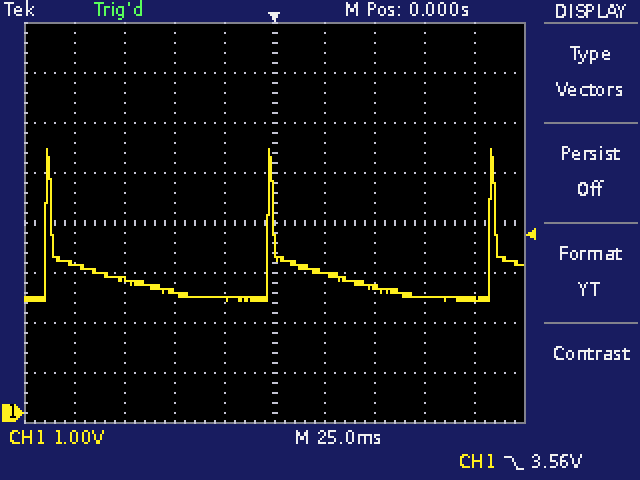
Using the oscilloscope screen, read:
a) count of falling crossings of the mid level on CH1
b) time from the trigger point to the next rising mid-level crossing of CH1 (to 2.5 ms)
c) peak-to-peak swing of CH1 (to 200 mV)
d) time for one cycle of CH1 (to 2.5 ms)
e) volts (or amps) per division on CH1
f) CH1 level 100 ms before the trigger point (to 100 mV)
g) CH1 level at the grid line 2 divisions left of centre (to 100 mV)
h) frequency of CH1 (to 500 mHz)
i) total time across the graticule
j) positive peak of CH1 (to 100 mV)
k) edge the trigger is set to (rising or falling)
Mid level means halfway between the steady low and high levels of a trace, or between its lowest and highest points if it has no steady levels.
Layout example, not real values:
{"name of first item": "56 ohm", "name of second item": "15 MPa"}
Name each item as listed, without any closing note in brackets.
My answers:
{"count of falling crossings of the mid level on CH1": "3", "time from the trigger point to the next rising mid-level crossing of CH1": "107.5 ms", "peak-to-peak swing of CH1": "3.0 V", "time for one cycle of CH1": "110.0 ms", "volts (or amps) per division on CH1": "1 V", "CH1 level 100 ms before the trigger point": "3.0 V", "CH1 level at the grid line 2 divisions left of centre": "2.4 V", "frequency of CH1": "9.0 Hz", "total time across the graticule": "250 ms", "positive peak of CH1": "5.3 V", "edge the trigger is set to": "falling"}
